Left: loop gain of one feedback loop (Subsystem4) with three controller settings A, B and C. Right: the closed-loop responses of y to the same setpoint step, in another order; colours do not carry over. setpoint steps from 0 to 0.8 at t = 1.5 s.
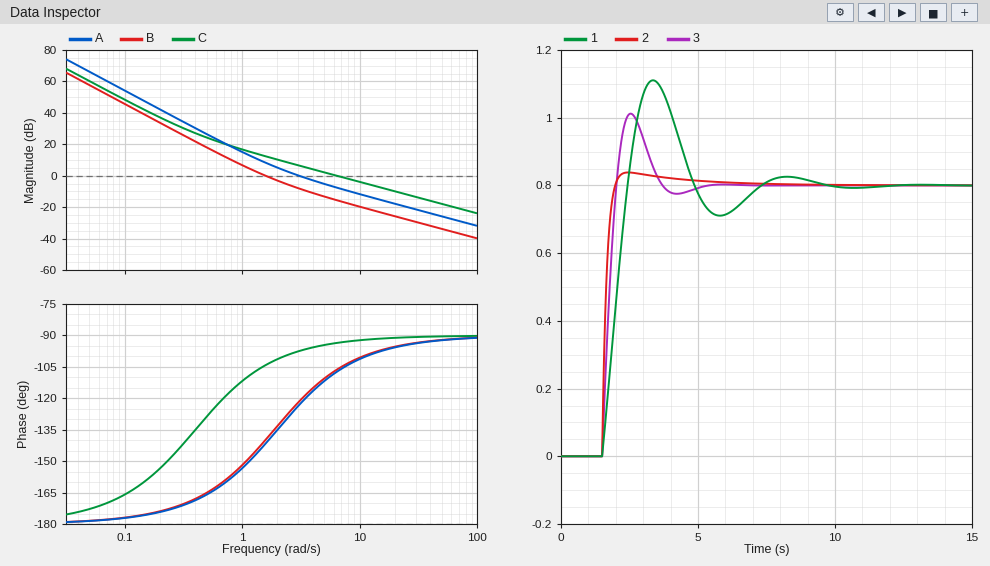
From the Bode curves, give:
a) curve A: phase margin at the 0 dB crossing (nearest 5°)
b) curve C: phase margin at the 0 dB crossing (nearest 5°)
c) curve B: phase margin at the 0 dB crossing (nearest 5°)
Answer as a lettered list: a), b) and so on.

a) 55°
b) 85°
c) 40°
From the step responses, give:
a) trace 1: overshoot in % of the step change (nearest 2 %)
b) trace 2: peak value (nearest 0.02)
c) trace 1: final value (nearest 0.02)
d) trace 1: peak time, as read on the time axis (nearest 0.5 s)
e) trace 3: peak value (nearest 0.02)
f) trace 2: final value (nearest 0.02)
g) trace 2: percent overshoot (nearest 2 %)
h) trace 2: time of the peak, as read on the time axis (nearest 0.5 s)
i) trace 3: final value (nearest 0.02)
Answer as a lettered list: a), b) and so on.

a) 38 %
b) 0.84
c) 0.80
d) 3.5 s
e) 1.02
f) 0.80
g) 4 %
h) 2.5 s
i) 0.80
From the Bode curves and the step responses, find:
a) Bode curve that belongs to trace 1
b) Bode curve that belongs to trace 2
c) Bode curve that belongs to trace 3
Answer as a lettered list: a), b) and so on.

a) B
b) C
c) A
